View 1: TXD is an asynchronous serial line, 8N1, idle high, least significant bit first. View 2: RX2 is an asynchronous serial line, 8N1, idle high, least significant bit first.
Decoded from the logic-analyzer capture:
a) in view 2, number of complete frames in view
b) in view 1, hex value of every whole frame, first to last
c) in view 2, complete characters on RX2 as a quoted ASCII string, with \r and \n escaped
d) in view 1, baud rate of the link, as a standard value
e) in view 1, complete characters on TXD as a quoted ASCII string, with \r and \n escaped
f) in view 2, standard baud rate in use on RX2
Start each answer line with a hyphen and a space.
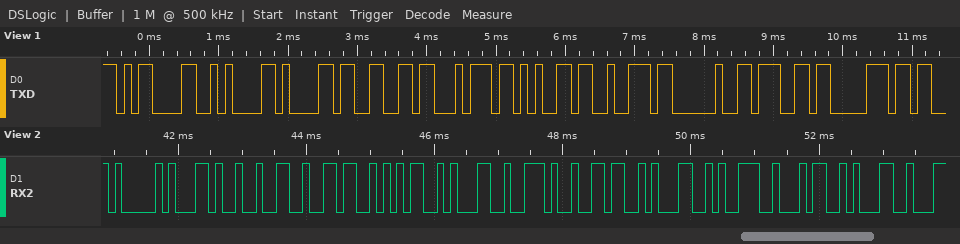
- 12
- 0D 0A 61 66 74 65 72 20 67 70
- "A,2651.61941"
- 9600 baud
- "\r\nafter gp"
- 9600 baud
